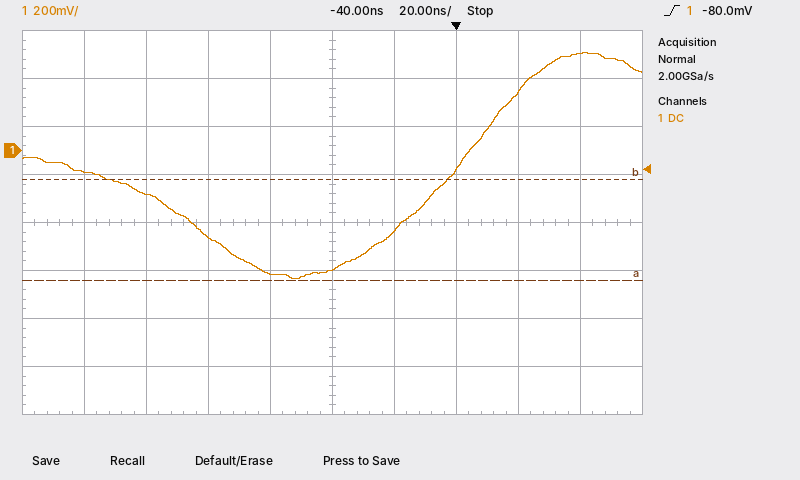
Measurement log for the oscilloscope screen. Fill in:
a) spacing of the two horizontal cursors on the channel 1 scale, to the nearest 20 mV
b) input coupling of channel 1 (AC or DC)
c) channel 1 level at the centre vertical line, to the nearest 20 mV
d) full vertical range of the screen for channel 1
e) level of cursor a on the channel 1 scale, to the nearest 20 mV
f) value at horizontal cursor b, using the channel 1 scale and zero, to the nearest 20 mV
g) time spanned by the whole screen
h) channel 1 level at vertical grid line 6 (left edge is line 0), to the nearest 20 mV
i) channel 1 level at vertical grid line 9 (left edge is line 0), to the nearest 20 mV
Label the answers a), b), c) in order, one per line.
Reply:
a) 420 mV
b) DC
c) -500 mV
d) 1.6 V
e) -540 mV
f) -120 mV
g) 200 ns
h) -340 mV
i) 400 mV
